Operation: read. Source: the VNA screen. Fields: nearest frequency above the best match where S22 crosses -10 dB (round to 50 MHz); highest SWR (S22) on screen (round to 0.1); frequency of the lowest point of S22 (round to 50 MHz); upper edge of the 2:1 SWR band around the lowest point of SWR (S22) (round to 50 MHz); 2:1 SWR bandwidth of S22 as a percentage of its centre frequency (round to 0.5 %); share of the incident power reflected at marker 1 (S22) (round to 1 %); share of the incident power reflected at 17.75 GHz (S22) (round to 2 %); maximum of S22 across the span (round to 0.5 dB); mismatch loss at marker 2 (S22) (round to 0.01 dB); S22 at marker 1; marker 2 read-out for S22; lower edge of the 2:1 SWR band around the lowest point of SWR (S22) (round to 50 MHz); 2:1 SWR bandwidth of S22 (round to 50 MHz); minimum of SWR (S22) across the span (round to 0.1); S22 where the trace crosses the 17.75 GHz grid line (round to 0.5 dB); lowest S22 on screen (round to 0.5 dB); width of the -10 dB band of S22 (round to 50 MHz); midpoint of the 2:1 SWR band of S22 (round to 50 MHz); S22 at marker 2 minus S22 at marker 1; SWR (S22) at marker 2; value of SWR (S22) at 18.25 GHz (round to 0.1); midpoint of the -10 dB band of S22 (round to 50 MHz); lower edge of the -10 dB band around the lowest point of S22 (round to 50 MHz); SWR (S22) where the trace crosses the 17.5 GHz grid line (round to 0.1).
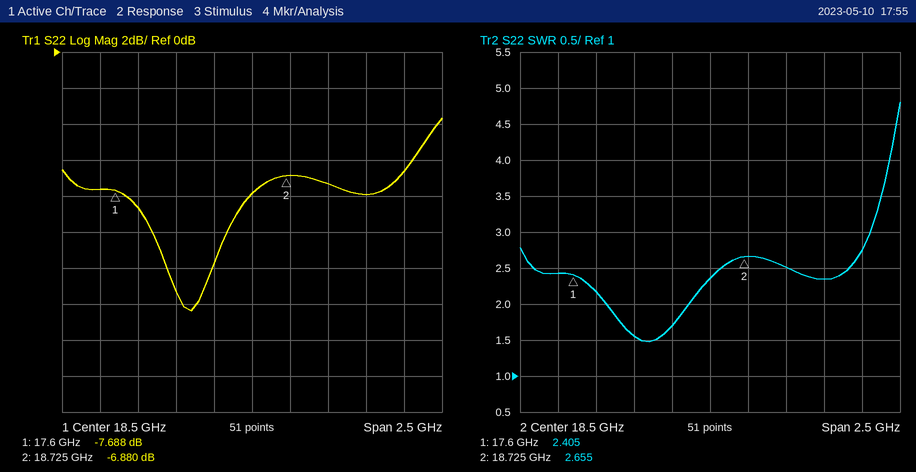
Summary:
18.35 GHz
4.8
18.10 GHz
18.35 GHz
3.0 %
17 %
14 %
-3.5 dB
1.00 dB
-7.688 dB
-6.880 dB
17.80 GHz
550 MHz
1.5
-8.5 dB
-14.5 dB
500 MHz
18.10 GHz
0.808 dB
2.655
1.7
18.10 GHz
17.85 GHz
2.4
